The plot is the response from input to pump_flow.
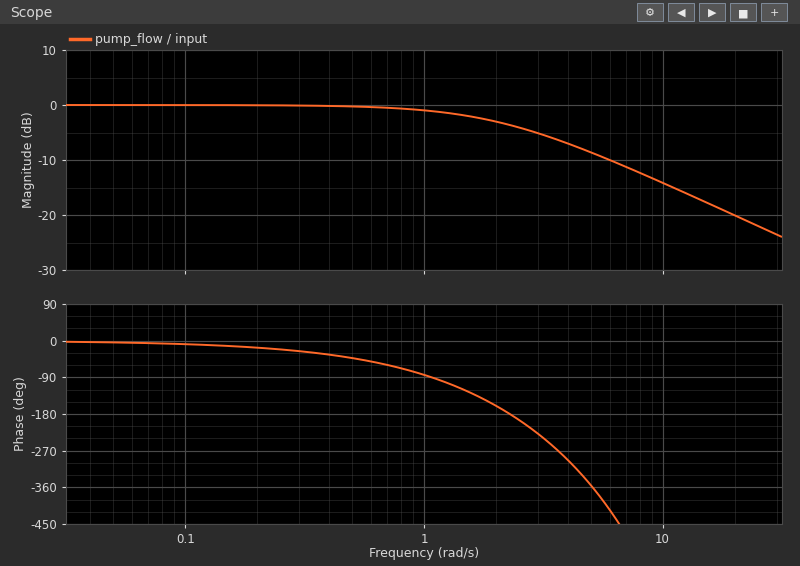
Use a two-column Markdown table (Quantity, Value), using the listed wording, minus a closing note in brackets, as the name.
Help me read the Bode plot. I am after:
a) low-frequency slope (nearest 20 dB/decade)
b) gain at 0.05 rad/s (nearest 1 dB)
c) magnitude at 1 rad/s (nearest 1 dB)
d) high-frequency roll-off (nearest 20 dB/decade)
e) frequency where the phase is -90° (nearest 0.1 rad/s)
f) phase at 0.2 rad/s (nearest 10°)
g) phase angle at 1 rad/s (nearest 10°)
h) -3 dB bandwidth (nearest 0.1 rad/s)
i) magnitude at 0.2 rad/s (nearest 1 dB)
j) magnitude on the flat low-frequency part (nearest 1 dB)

| Quantity | Value |
|---|---|
| low-frequency slope | 0 dB/decade |
| gain at 0.05 rad/s | 0 dB |
| magnitude at 1 rad/s | -1 dB |
| high-frequency roll-off | -20 dB/decade |
| frequency where the phase is -90° | 1.1 rad/s |
| phase at 0.2 rad/s | -20° |
| phase angle at 1 rad/s | -80° |
| -3 dB bandwidth | 2.0 rad/s |
| magnitude at 0.2 rad/s | 0 dB |
| magnitude on the flat low-frequency part | 0 dB |
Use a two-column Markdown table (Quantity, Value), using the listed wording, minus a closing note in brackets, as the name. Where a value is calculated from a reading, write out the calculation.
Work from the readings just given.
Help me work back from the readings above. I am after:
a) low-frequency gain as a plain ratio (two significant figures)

| Quantity | Value |
|---|---|
| low-frequency gain as a plain ratio | 10^(0 / 20) = 1.0 |
